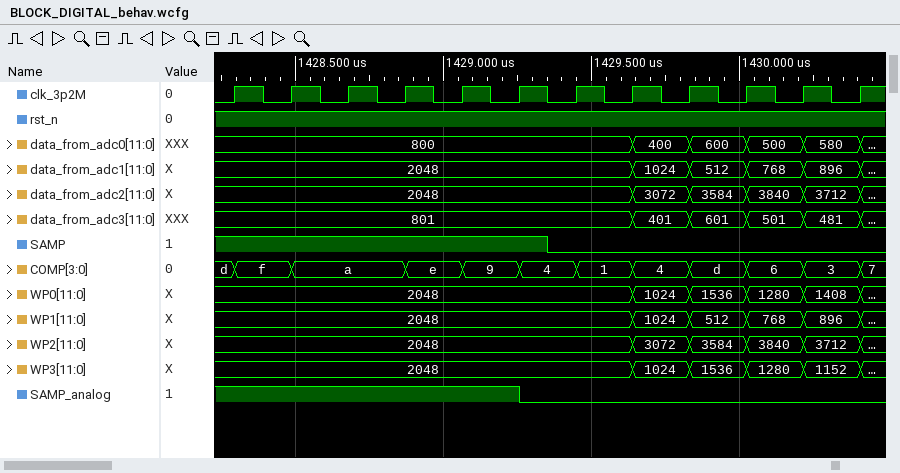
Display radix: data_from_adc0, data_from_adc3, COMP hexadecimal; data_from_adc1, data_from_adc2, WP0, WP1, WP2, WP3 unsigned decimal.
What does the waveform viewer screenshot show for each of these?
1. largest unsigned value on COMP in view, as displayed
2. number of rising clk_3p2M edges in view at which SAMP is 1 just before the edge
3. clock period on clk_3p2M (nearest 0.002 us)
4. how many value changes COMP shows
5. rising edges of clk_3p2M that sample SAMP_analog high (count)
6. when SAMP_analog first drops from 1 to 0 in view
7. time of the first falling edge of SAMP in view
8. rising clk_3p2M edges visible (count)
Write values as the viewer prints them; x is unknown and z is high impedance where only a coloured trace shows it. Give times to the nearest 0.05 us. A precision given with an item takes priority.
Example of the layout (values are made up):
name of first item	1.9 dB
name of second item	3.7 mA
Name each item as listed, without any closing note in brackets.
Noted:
largest unsigned value on COMP in view, as displayed	f
number of rising clk_3p2M edges in view at which SAMP is 1 just before the edge	6
clock period on clk_3p2M	0.192 us
how many value changes COMP shows	11
rising edges of clk_3p2M that sample SAMP_analog high	6
when SAMP_analog first drops from 1 to 0 in view	1429.25 us
time of the first falling edge of SAMP in view	1429.35 us
rising clk_3p2M edges visible	12
